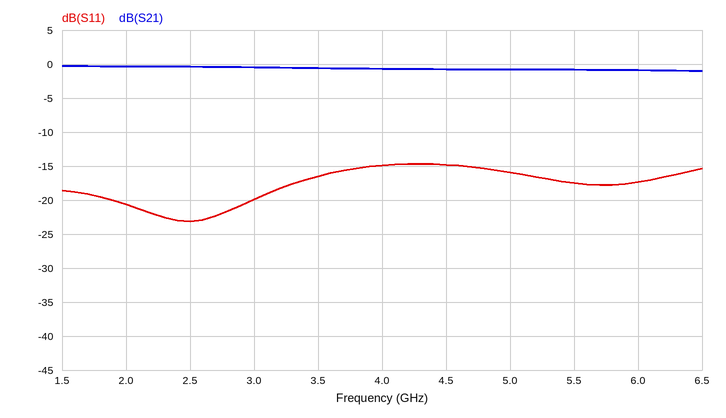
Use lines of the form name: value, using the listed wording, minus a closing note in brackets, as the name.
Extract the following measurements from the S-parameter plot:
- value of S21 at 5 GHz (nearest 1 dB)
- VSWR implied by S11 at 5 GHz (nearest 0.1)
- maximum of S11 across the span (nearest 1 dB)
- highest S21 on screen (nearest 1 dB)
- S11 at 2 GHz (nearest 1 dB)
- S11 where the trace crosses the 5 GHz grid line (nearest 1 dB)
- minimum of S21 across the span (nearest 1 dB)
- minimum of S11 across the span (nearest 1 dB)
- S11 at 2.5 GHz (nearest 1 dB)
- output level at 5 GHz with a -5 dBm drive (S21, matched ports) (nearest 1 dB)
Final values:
value of S21 at 5 GHz: -1 dB
VSWR implied by S11 at 5 GHz: 1.4
maximum of S11 across the span: -15 dB
highest S21 on screen: 0 dB
S11 at 2 GHz: -21 dB
S11 where the trace crosses the 5 GHz grid line: -16 dB
minimum of S21 across the span: -1 dB
minimum of S11 across the span: -23 dB
S11 at 2.5 GHz: -23 dB
output level at 5 GHz with a -5 dBm drive (S21, matched ports): -6 dBm
